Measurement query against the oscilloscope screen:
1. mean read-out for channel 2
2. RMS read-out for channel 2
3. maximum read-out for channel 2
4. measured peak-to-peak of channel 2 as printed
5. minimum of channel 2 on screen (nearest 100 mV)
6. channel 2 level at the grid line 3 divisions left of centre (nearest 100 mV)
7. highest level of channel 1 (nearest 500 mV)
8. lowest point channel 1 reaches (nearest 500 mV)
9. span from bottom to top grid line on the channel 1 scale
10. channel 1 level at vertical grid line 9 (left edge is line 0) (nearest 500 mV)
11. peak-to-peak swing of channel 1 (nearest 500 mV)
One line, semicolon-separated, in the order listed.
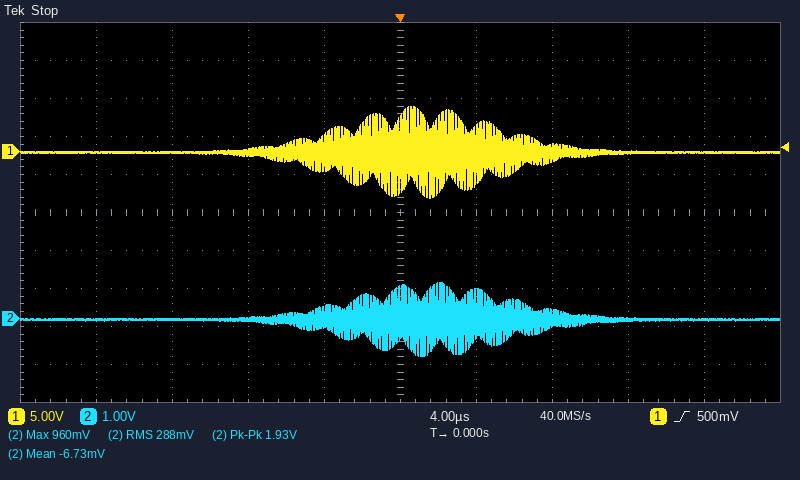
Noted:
-6.73 mV; 288 mV; 960 mV; 1.93 V; -1.0 V; 0.0 V; 6.0 V; -6.0 V; 50 V; 0.0 V; 12.0 V
